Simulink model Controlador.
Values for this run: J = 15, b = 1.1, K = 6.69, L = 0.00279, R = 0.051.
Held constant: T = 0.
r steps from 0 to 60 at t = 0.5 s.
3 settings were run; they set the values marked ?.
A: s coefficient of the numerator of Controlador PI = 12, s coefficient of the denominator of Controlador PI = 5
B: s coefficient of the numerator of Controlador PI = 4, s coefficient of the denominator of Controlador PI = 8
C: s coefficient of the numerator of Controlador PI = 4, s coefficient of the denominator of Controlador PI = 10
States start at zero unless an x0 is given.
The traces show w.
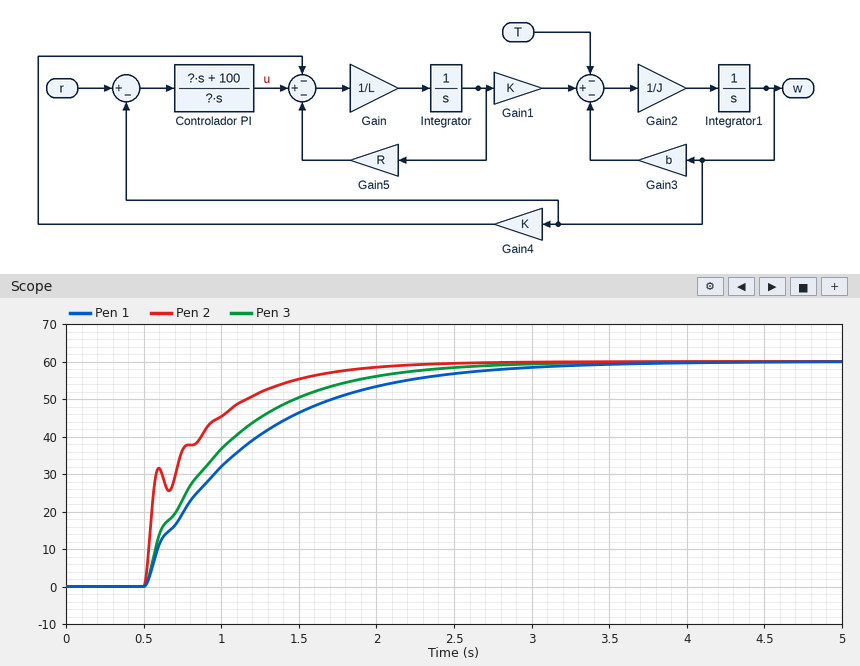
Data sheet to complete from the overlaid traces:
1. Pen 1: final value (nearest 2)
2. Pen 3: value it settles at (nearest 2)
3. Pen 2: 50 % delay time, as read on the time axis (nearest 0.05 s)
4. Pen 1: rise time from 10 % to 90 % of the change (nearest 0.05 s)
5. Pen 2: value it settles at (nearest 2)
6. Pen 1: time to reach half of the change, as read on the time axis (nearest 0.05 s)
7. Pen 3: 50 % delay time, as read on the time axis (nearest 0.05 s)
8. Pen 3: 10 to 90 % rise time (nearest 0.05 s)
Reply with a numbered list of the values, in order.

1. 60
2. 60
3. 0.60 s
4. 1.50 s
5. 60
6. 0.95 s
7. 0.85 s
8. 1.20 s
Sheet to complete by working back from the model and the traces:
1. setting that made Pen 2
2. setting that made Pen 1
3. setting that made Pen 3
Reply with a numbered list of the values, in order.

1. A
2. C
3. B
